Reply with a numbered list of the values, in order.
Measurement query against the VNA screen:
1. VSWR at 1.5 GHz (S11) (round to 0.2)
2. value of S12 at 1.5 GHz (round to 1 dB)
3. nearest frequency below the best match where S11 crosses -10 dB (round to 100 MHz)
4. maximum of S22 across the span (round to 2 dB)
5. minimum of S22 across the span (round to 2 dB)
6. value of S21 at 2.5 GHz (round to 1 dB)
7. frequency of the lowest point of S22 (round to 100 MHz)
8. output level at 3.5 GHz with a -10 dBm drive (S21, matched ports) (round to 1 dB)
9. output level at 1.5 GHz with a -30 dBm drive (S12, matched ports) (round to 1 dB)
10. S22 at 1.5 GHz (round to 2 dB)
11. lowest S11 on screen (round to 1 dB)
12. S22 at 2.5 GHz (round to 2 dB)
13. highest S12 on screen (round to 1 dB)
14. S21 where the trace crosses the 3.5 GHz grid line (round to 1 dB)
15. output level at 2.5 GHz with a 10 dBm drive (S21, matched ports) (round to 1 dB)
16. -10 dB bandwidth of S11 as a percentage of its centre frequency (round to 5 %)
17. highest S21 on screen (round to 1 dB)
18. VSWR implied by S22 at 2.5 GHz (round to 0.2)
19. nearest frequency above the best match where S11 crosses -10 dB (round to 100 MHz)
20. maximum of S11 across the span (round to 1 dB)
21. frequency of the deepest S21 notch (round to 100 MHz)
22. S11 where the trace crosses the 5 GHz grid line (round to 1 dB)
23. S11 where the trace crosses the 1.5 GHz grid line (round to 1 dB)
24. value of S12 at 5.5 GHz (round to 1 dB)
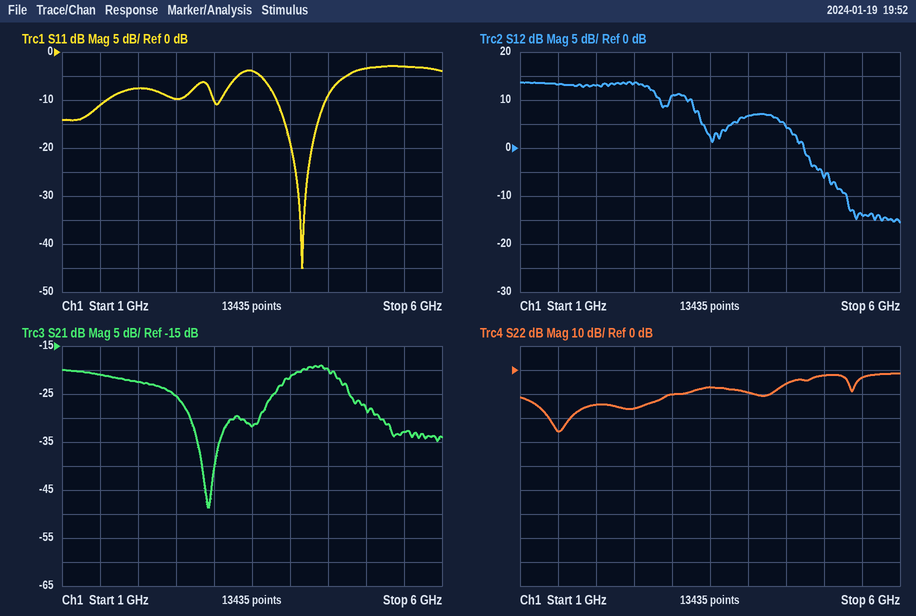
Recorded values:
1. 1.8
2. 13 dB
3. 3.8 GHz
4. -2 dB
5. -26 dB
6. -25 dB
7. 1.5 GHz
8. -42 dBm
9. -17 dBm
10. -26 dB
11. -45 dB
12. -16 dB
13. 14 dB
14. -32 dB
15. -15 dBm
16. 15 %
17. -19 dB
18. 1.4
19. 4.5 GHz
20. -3 dB
21. 2.9 GHz
22. -3 dB
23. -11 dB
24. -14 dB
